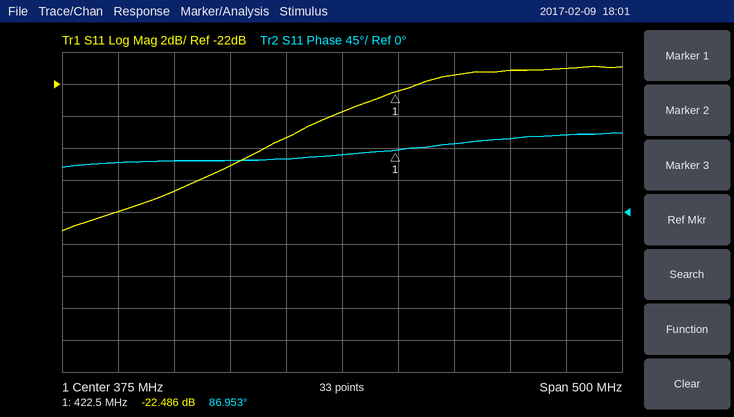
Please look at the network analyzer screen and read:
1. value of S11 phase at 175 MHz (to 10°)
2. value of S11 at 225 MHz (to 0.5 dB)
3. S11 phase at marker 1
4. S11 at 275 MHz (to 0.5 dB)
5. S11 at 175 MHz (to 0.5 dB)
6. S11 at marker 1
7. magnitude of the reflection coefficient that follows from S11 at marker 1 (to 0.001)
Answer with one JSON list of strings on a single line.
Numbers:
["70°", "-28.5 dB", "86.953°", "-27.0 dB", "-30.0 dB", "-22.486 dB", "0.075"]
